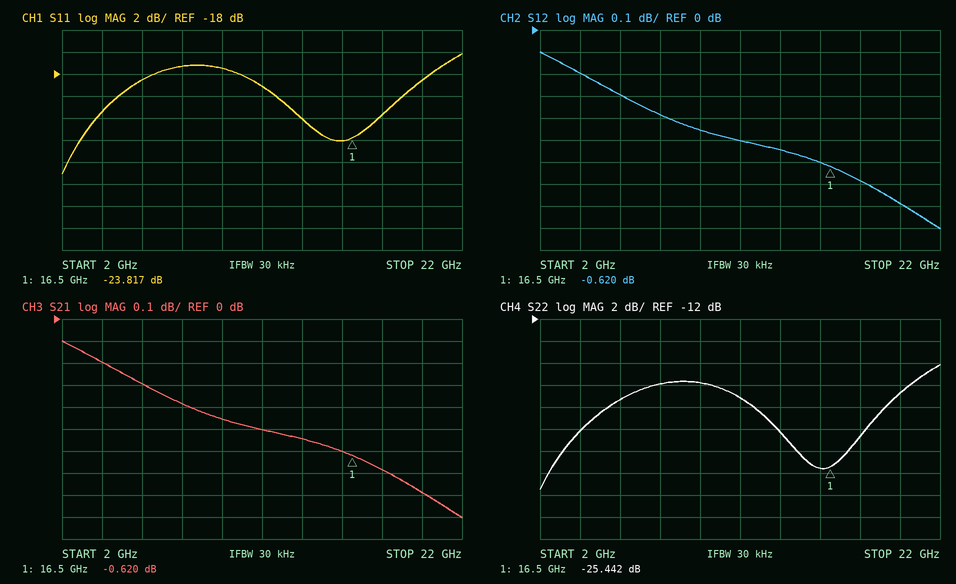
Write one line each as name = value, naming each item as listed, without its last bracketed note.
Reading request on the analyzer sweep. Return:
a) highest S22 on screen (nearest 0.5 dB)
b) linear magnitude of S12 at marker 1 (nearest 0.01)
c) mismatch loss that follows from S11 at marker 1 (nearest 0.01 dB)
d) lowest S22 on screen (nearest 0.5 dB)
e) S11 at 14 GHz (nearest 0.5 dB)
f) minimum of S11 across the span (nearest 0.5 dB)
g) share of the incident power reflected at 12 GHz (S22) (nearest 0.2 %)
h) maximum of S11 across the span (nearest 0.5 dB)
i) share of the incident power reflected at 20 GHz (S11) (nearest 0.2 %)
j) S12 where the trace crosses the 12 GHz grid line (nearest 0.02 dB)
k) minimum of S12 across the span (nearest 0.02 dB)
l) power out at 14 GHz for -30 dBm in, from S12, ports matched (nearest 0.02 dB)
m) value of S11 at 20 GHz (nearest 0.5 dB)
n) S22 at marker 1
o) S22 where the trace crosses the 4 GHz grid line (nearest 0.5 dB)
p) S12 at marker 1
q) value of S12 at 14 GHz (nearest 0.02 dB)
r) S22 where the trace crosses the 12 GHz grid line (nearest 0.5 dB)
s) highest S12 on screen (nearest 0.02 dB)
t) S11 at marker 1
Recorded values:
highest S22 on screen = -16.0 dB
linear magnitude of S12 at marker 1 = 0.93
mismatch loss that follows from S11 at marker 1 = 0.02 dB
lowest S22 on screen = -27.5 dB
S11 at 14 GHz = -22.0 dB
minimum of S11 across the span = -27.0 dB
share of the incident power reflected at 12 GHz (S22) = 1.2 %
maximum of S11 across the span = -16.0 dB
share of the incident power reflected at 20 GHz (S11) = 1.4 %
S12 where the trace crosses the 12 GHz grid line = -0.50 dB
minimum of S12 across the span = -0.90 dB
power out at 14 GHz for -30 dBm in, from S12, ports matched = -30.54 dBm
value of S11 at 20 GHz = -18.5 dB
S22 at marker 1 = -25.442 dB
S22 where the trace crosses the 4 GHz grid line = -22.0 dB
S12 at marker 1 = -0.620 dB
value of S12 at 14 GHz = -0.54 dB
S22 where the trace crosses the 12 GHz grid line = -19.0 dB
highest S12 on screen = -0.10 dB
S11 at marker 1 = -23.817 dB
